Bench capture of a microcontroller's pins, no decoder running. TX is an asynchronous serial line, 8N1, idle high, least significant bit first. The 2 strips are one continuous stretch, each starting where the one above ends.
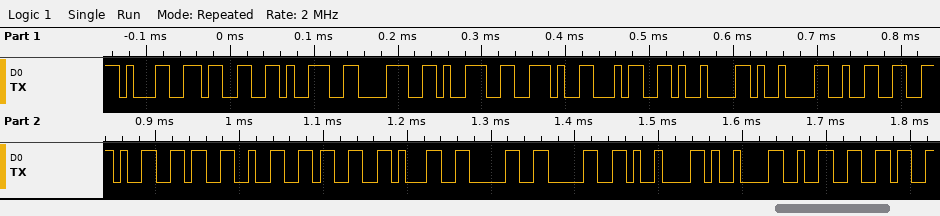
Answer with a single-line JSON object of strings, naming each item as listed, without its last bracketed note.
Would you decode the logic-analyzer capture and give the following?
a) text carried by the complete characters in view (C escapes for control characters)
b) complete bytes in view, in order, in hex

{"text carried by the complete characters in view": "\"13989.4\\t\\t2.623100\\t\\t26\"", "complete bytes in view, in order, in hex": "0x31 0x33 0x39 0x38 0x39 0x2E 0x34 0x09 0x09 0x32 0x2E 0x36 0x32 0x33 0x31 0x30 0x30 0x09 0x09 0x32 0x36"}
